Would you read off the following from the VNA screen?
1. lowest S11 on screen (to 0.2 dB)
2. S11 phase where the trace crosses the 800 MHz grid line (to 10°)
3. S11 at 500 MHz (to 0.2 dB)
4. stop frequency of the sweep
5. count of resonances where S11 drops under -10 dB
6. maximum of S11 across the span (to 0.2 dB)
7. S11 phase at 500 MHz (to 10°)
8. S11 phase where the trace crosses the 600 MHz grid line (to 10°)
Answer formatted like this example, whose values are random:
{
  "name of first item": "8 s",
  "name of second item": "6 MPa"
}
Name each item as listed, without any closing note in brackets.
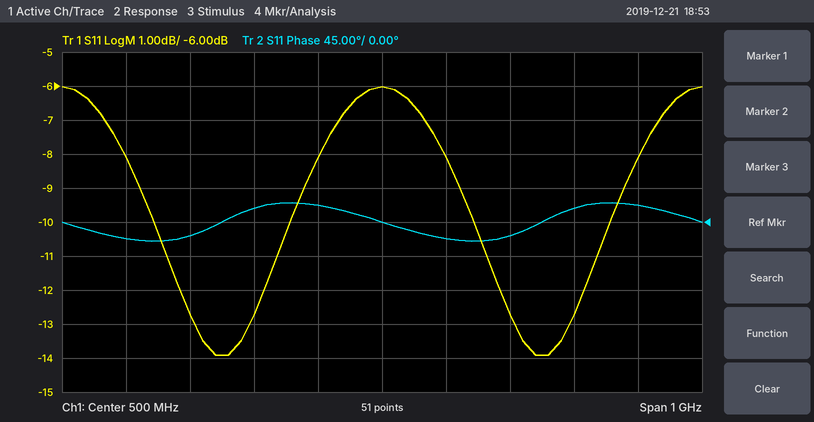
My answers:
{
  "lowest S11 on screen": "-14.0 dB",
  "S11 phase where the trace crosses the 800 MHz grid line": "20°",
  "S11 at 500 MHz": "-6.0 dB",
  "stop frequency of the sweep": "1 GHz",
  "count of resonances where S11 drops under -10 dB": "2",
  "maximum of S11 across the span": "-6.0 dB",
  "S11 phase at 500 MHz": "0°",
  "S11 phase where the trace crosses the 600 MHz grid line": "-20°"
}
